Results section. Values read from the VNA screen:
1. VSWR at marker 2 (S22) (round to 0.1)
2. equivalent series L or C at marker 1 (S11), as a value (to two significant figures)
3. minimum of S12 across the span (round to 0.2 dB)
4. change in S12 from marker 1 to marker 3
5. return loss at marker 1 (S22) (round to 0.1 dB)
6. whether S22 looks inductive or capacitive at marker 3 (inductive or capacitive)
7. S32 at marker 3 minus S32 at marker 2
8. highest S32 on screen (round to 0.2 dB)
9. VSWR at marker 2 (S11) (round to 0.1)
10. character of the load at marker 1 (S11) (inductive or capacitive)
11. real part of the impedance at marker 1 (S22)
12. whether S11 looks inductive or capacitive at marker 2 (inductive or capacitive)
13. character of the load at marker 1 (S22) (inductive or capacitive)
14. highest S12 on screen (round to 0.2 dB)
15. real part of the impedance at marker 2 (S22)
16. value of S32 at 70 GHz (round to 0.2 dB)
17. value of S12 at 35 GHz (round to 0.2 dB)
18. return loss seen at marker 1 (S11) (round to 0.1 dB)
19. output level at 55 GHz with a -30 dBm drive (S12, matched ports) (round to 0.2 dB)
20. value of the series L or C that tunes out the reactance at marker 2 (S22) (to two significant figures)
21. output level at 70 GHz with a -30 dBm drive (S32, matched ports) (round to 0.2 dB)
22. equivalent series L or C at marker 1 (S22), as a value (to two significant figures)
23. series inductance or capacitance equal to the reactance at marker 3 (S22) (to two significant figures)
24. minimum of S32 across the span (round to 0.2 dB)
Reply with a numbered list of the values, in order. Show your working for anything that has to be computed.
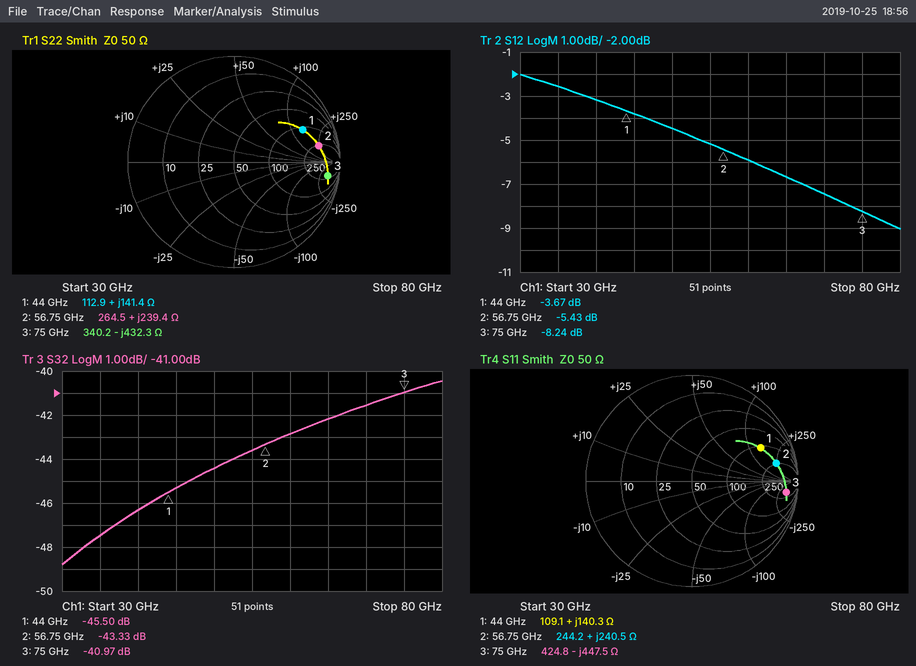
1. 9.7
2. L = 140.3 Ω/(2π × 44 GHz) ≈ 507 pH, so 510 pH to two significant figures
3. -9.0 dB
4. -8.24 − (-3.67) = -4.57 dB
5. 2.9 dB
6. capacitive
7. -40.97 − (-43.33) = 2.36 dB
8. -40.4 dB
9. 9.7
10. inductive
11. 112.9 Ω
12. inductive
13. inductive
14. -2.0 dB
15. 264.5 Ω
16. -41.6 dB
17. -2.6 dB
18. 2.9 dB
19. -30 dBm + (-5.2 dB) = -35.2 dBm
20. C = 1/(2π × 56.75 GHz × 239.4 Ω) ≈ 12 fF
21. -30 dBm + (-41.6 dB) = -71.6 dBm
22. L = 141.4 Ω/(2π × 44 GHz) ≈ 511 pH, so 510 pH to two significant figures
23. C = 1/(2π × 75 GHz × 432.3 Ω) ≈ 4.9 fF
24. -48.8 dB
